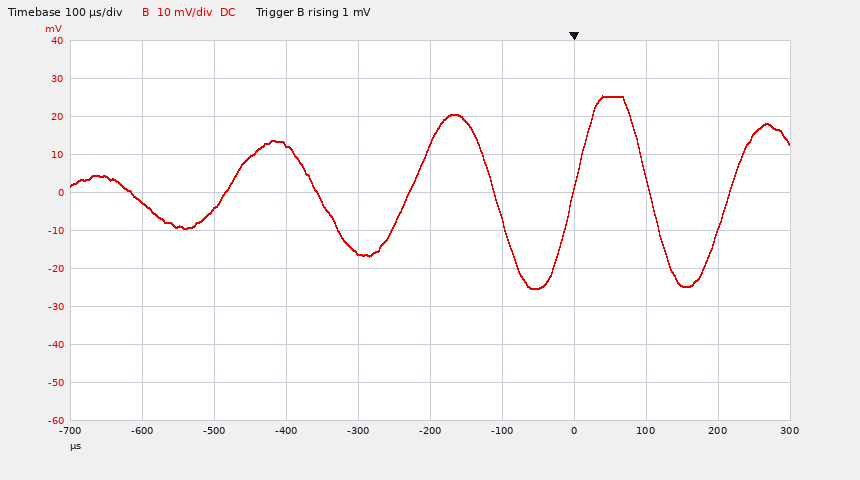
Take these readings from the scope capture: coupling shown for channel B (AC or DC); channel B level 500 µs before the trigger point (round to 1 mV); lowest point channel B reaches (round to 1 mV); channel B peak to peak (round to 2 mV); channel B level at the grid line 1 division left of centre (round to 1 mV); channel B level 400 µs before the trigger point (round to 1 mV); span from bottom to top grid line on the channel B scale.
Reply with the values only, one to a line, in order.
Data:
DC
-4 mV
-25 mV
50 mV
-16 mV
13 mV
100 mV
